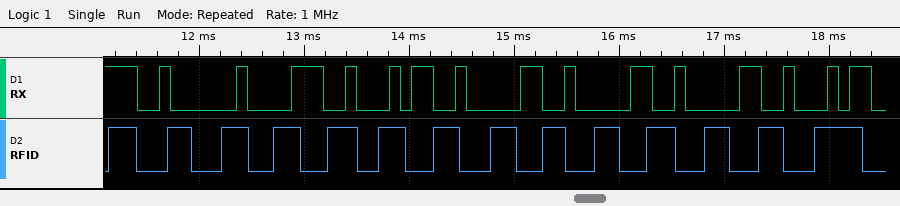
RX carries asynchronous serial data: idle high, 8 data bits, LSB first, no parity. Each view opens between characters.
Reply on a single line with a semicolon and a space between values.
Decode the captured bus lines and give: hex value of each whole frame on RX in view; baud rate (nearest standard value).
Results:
02, 38, 34, 30, 30, 30; 9600 baud
